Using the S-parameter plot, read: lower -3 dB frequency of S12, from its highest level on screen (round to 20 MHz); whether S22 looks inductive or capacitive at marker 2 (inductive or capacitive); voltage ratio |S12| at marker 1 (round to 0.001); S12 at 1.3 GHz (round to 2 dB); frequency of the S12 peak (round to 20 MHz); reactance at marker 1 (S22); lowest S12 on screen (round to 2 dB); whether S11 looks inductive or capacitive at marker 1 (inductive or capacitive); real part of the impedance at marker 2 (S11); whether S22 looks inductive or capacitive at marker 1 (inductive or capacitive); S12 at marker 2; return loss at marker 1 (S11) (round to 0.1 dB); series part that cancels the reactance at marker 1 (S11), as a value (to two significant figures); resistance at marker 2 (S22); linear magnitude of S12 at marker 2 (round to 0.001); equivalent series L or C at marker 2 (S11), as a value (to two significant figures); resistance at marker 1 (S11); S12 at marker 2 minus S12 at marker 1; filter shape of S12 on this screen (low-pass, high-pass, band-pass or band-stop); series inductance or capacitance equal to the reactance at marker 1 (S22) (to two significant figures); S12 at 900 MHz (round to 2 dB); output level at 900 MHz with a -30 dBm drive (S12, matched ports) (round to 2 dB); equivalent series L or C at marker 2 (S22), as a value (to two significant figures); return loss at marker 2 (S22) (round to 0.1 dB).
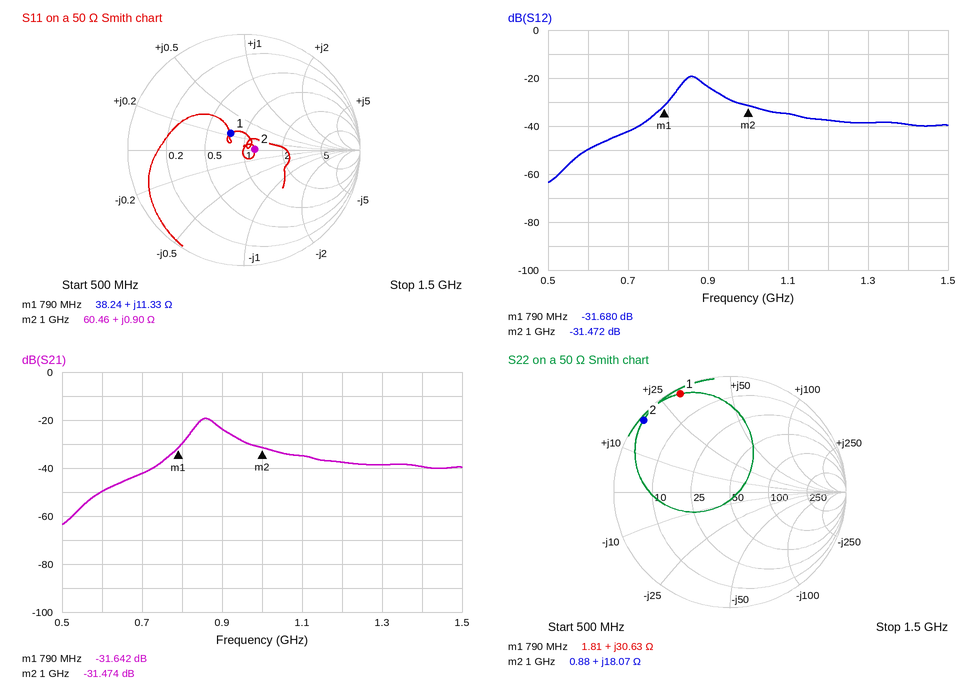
840 MHz
inductive
0.026
-38 dB
860 MHz
+30.63 Ω
-64 dB
inductive
60.46 Ω
inductive
-31.472 dB
14.7 dB
18 pF
0.88 Ω
0.027
140 pH
38.24 Ω
0.208 dB
band-pass
6.2 nH
-24 dB
-54 dBm
2.9 nH
0.3 dB
